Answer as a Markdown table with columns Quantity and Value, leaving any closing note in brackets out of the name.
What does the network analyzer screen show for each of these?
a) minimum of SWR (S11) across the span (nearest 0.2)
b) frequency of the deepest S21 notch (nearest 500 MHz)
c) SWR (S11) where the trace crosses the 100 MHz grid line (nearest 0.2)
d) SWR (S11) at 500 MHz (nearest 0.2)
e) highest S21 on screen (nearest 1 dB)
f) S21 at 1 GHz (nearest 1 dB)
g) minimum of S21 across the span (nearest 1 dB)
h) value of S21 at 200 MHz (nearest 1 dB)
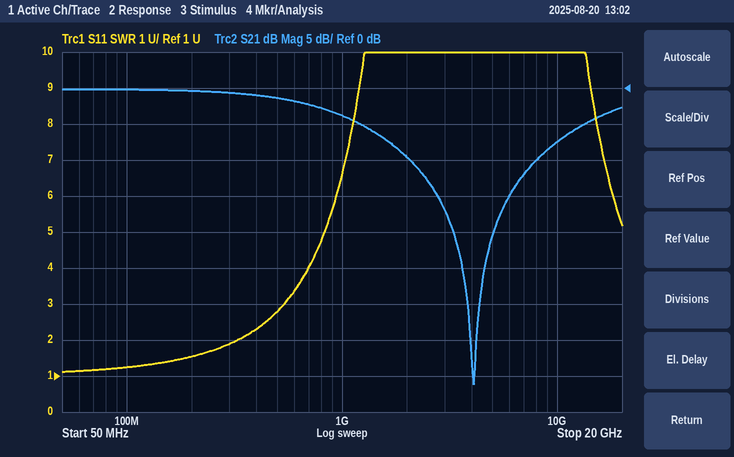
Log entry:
| Quantity | Value |
|---|---|
| minimum of SWR (S11) across the span | 1.2 |
| frequency of the deepest S21 notch | 4.0 GHz |
| SWR (S11) where the trace crosses the 100 MHz grid line | 1.2 |
| SWR (S11) at 500 MHz | 2.8 |
| highest S21 on screen | 0 dB |
| S21 at 1 GHz | -4 dB |
| minimum of S21 across the span | -41 dB |
| value of S21 at 200 MHz | 0 dB |
